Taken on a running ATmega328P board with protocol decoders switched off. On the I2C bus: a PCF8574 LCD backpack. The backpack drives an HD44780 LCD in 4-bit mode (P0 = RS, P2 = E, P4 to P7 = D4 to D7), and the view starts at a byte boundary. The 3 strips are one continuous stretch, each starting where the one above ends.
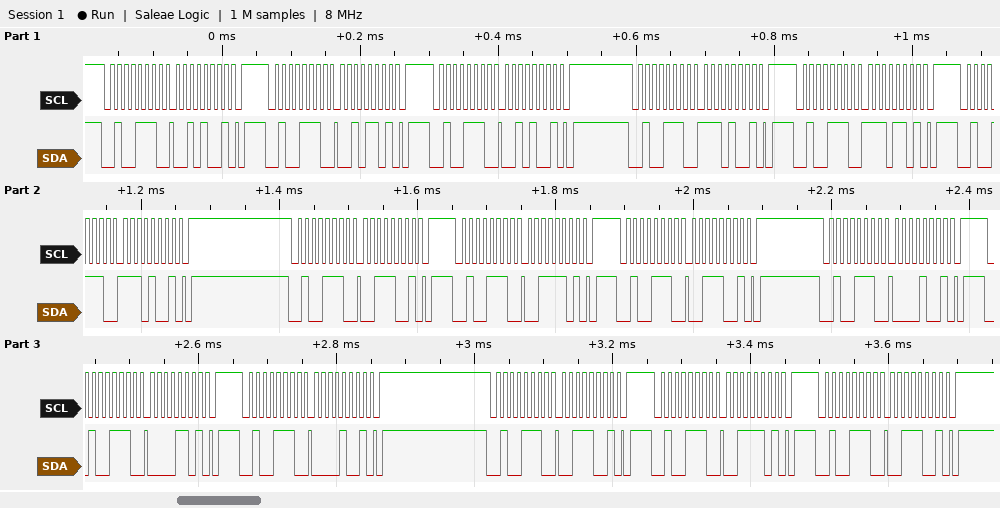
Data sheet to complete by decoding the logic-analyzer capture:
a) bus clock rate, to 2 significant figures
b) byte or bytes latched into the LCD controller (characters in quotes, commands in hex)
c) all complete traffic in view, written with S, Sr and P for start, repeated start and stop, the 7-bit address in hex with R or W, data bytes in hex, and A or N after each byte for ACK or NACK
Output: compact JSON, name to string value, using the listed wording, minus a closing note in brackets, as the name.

{"bus clock rate, to 2 significant figures": "100 kHz", "byte or bytes latched into the LCD controller": "'.' '0'", "all complete traffic in view, written with S, Sr and P for start, repeated start and stop, the 7-bit address in hex with R or W, data bytes in hex, and A or N after each byte for ACK or NACK": "S 27W A 29 A P S 27W A 2D A P S 27W A 29 A P S 27W A E9 A P S 27W A ED A P S 27W A E9 A P S 27W A 39 A P S 27W A 3D A P S 27W A 39 A P S 27W A 09 A P S 27W A 0D A P S 27W A 09 A P S 27W A 39 A P S 27W A 3D A P S 27W A 39 A P"}
